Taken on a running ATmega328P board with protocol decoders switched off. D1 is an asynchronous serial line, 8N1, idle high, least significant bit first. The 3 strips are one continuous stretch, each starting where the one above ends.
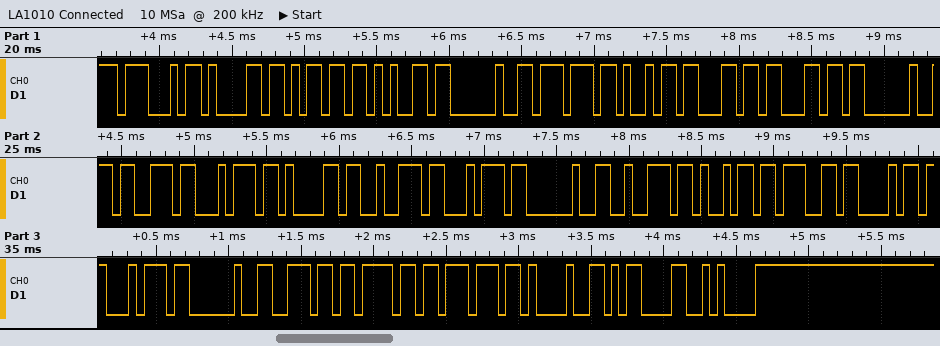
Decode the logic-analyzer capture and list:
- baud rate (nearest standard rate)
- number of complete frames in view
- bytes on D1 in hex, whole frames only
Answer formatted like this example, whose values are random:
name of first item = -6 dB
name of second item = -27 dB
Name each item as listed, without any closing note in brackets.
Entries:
baud rate = 19200 baud
number of complete frames in view = 28
bytes on D1 in hex, whole frames only = 47 61 6D 65 20 77 69 6C 6C 20 73 74 61 72 74 20 72 69 67 68 74 20 6E 6F 77 21 0D 0A
